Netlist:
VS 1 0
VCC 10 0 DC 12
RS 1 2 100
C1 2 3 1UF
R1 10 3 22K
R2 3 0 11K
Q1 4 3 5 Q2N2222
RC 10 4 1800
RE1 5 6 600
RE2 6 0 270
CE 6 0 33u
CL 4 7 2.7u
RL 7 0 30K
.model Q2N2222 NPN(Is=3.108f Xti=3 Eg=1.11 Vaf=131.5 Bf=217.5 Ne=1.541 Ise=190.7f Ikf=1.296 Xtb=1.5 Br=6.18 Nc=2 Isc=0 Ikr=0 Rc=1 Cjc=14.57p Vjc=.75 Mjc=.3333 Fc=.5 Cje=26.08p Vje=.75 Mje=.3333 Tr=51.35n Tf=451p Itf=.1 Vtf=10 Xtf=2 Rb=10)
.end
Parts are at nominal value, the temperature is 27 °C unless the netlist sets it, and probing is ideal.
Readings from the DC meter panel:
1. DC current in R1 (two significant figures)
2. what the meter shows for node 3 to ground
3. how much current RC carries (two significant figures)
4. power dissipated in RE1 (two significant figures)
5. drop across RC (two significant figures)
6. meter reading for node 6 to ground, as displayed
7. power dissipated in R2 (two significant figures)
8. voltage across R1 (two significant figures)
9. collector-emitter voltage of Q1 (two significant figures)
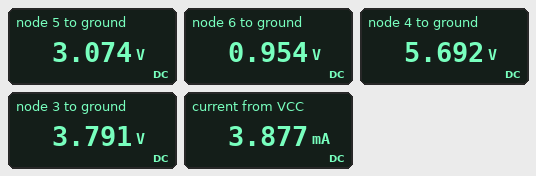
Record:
370 µA
3.791 V
3.5 mA
7.5 mW
6.3 V
0.954 V
1.3 mW
8.2 V
2.6 V
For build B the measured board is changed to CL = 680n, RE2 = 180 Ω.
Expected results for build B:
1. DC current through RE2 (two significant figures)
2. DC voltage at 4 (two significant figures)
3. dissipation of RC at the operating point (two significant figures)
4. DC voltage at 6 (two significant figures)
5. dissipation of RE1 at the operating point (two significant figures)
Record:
3.9 mA
5.0 V
27 mW
700 mV
9.2 mW
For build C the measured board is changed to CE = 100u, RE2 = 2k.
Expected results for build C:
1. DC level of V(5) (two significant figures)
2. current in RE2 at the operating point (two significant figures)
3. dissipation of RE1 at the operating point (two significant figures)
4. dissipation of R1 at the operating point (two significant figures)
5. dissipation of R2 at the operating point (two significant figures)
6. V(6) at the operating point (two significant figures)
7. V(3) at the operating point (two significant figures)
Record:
3.2 V
1.2 mA
920 µW
3.0 mW
1.4 mW
2.5 V
3.9 V
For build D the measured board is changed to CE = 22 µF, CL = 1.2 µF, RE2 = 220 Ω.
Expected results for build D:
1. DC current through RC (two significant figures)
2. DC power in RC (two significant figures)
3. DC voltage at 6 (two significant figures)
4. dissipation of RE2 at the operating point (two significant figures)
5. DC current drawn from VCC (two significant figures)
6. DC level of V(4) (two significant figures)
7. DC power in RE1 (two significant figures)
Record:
3.7 mA
25 mW
820 mV
3.1 mW
4.1 mA
5.3 V
8.4 mW
